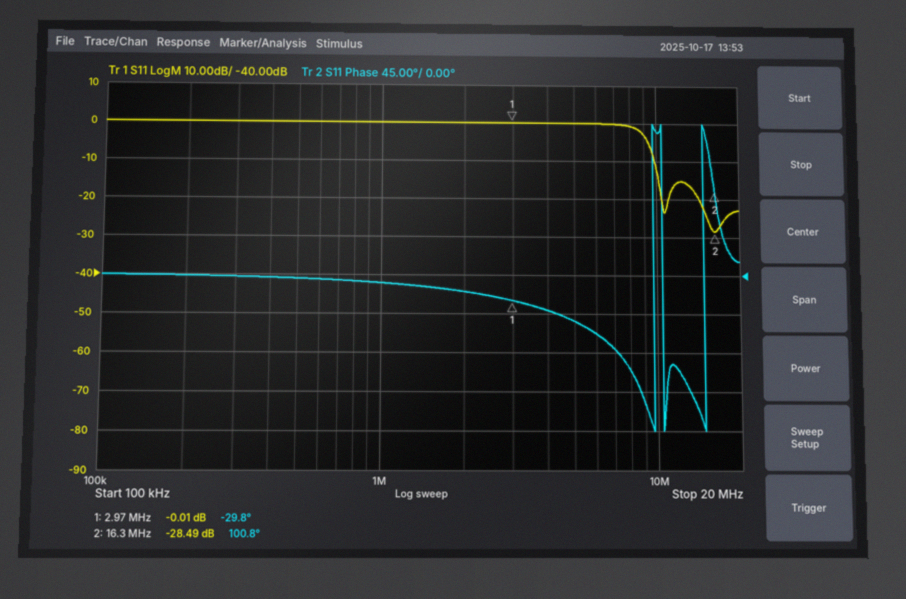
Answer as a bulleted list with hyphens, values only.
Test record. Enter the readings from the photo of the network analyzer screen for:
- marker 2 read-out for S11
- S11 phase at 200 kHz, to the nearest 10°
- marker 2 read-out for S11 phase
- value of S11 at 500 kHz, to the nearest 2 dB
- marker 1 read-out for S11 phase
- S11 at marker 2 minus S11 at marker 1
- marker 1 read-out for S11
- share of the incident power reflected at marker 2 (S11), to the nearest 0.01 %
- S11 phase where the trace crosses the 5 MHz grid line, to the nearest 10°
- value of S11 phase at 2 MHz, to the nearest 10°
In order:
- -28.49 dB
- 0°
- 100.8°
- 0 dB
- -29.8°
- -28.48 dB
- -0.01 dB
- 0.14 %
- -50°
- -20°
